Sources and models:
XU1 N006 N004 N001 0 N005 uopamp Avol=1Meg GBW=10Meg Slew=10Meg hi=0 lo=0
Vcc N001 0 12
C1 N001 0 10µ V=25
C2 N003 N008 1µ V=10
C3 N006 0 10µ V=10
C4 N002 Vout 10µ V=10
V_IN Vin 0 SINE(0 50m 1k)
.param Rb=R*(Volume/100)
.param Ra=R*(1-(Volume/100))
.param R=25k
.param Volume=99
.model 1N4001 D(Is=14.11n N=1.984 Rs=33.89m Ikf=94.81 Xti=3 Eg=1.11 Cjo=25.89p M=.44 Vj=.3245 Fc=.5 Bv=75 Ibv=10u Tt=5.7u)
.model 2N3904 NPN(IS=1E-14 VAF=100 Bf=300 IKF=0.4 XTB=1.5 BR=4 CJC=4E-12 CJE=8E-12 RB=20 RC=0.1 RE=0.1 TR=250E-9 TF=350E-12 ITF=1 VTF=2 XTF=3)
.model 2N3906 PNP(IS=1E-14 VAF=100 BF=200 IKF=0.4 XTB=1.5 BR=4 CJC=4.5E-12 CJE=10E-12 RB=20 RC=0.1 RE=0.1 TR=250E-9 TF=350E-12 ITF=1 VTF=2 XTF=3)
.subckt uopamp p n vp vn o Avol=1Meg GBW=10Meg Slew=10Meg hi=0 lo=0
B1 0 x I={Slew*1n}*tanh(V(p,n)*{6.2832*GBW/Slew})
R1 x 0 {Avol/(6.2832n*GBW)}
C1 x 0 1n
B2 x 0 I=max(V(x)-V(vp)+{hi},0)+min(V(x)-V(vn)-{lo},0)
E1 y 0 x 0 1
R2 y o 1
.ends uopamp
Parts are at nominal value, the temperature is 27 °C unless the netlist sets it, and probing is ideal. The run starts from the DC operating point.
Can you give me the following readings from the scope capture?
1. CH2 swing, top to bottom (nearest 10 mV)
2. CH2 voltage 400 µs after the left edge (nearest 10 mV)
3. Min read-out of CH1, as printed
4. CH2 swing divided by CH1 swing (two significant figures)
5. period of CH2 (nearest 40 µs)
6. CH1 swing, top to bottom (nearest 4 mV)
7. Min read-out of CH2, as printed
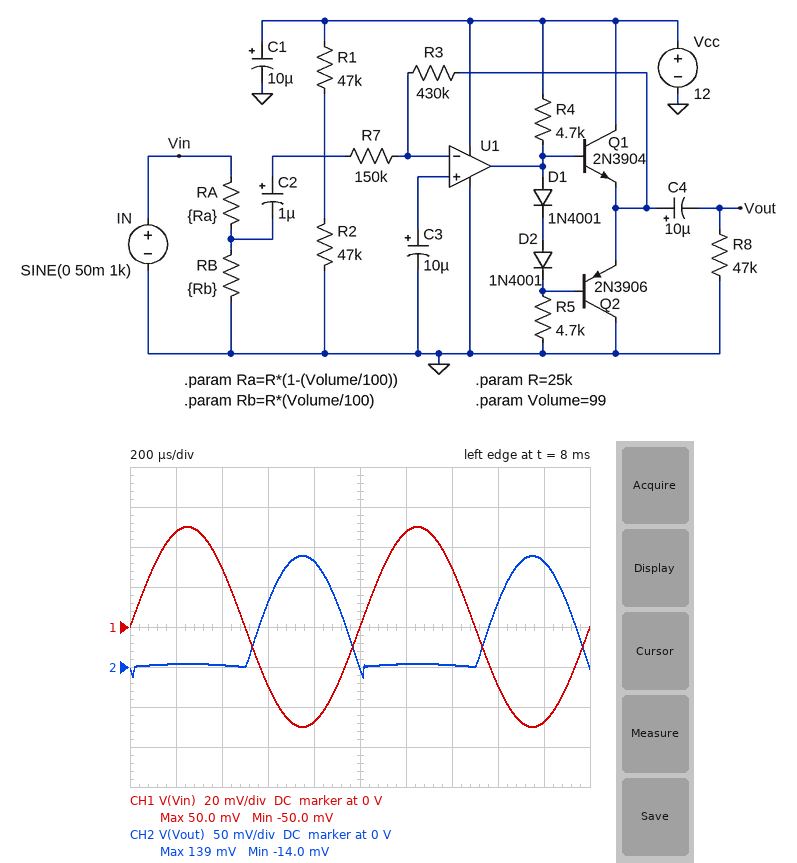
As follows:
150 mV
0 V
-50.0 mV
1.5
1.00 ms
100 mV
-14.0 mV
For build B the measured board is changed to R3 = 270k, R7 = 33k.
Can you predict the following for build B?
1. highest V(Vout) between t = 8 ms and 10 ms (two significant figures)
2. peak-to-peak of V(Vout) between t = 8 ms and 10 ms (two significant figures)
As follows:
370 mV
390 mV
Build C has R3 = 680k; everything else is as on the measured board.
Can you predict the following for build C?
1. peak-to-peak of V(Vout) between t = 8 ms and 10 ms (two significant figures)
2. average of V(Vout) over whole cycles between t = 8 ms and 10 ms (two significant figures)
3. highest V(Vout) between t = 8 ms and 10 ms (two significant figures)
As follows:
240 mV
70 mV
220 mV
